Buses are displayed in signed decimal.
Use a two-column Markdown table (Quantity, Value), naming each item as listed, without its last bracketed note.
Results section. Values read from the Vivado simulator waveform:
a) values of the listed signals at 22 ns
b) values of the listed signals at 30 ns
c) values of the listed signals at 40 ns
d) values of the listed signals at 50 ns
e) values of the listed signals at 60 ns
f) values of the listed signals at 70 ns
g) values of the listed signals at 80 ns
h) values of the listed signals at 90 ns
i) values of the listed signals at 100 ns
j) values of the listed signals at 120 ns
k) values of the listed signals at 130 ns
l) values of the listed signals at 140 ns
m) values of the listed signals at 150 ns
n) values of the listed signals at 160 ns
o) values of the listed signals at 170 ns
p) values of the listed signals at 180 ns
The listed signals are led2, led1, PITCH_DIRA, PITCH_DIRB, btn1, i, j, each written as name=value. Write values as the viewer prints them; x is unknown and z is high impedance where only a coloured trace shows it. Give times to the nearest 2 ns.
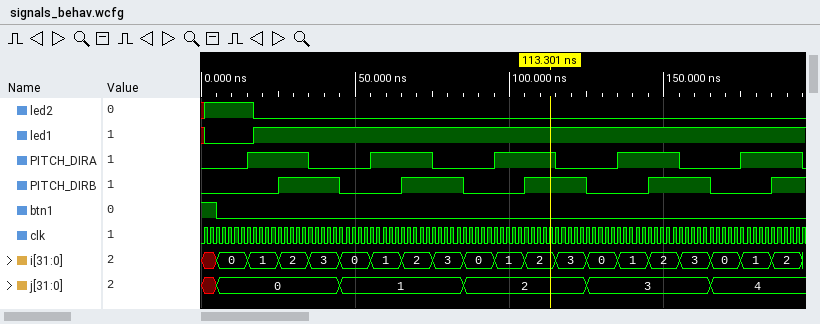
| Quantity | Value |
|---|---|
| values of the listed signals at 22 ns | led2=0, led1=1, PITCH_DIRA=1, PITCH_DIRB=0, btn1=0, i=1, j=0 |
| values of the listed signals at 30 ns | led2=0, led1=1, PITCH_DIRA=1, PITCH_DIRB=1, btn1=0, i=2, j=0 |
| values of the listed signals at 40 ns | led2=0, led1=1, PITCH_DIRA=0, PITCH_DIRB=1, btn1=0, i=3, j=0 |
| values of the listed signals at 50 ns | led2=0, led1=1, PITCH_DIRA=0, PITCH_DIRB=0, btn1=0, i=0, j=1 |
| values of the listed signals at 60 ns | led2=0, led1=1, PITCH_DIRA=1, PITCH_DIRB=0, btn1=0, i=1, j=1 |
| values of the listed signals at 70 ns | led2=0, led1=1, PITCH_DIRA=1, PITCH_DIRB=1, btn1=0, i=2, j=1 |
| values of the listed signals at 80 ns | led2=0, led1=1, PITCH_DIRA=0, PITCH_DIRB=1, btn1=0, i=3, j=1 |
| values of the listed signals at 90 ns | led2=0, led1=1, PITCH_DIRA=0, PITCH_DIRB=0, btn1=0, i=0, j=2 |
| values of the listed signals at 100 ns | led2=0, led1=1, PITCH_DIRA=1, PITCH_DIRB=0, btn1=0, i=1, j=2 |
| values of the listed signals at 120 ns | led2=0, led1=1, PITCH_DIRA=0, PITCH_DIRB=1, btn1=0, i=3, j=2 |
| values of the listed signals at 130 ns | led2=0, led1=1, PITCH_DIRA=0, PITCH_DIRB=0, btn1=0, i=0, j=3 |
| values of the listed signals at 140 ns | led2=0, led1=1, PITCH_DIRA=1, PITCH_DIRB=0, btn1=0, i=1, j=3 |
| values of the listed signals at 150 ns | led2=0, led1=1, PITCH_DIRA=1, PITCH_DIRB=1, btn1=0, i=2, j=3 |
| values of the listed signals at 160 ns | led2=0, led1=1, PITCH_DIRA=0, PITCH_DIRB=1, btn1=0, i=3, j=3 |
| values of the listed signals at 170 ns | led2=0, led1=1, PITCH_DIRA=0, PITCH_DIRB=0, btn1=0, i=0, j=4 |
| values of the listed signals at 180 ns | led2=0, led1=1, PITCH_DIRA=1, PITCH_DIRB=0, btn1=0, i=1, j=4 |
